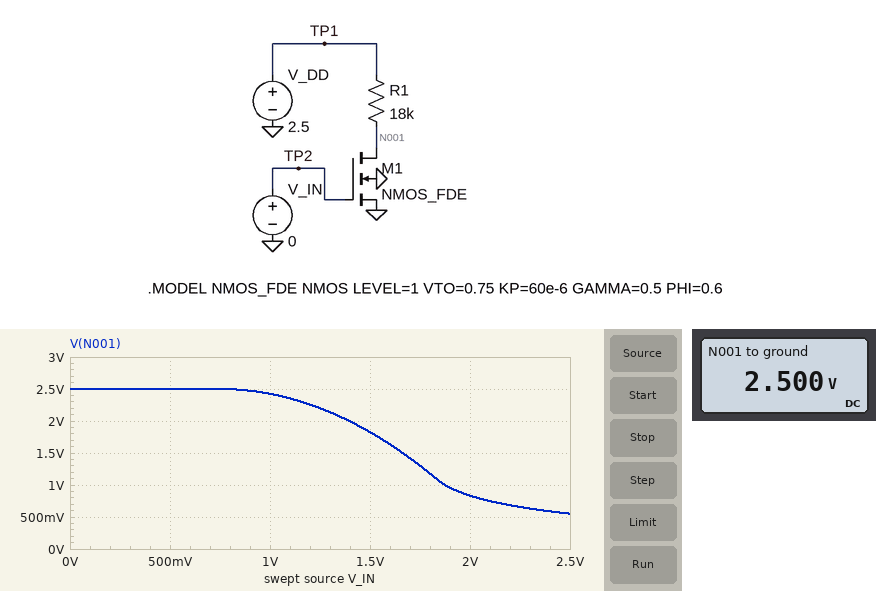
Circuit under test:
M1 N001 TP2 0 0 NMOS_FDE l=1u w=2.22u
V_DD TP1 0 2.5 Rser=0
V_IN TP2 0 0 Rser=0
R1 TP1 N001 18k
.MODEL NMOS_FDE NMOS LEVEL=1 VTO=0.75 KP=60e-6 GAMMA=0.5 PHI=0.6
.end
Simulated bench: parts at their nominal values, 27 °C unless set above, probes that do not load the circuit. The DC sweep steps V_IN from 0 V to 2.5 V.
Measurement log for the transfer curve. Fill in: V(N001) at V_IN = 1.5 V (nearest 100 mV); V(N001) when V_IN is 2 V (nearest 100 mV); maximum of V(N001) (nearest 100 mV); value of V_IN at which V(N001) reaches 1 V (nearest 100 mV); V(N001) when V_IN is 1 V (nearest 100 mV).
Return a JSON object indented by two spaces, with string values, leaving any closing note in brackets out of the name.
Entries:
{
  "V(N001) at V_IN = 1.5 V": "1.8 V",
  "V(N001) when V_IN is 2 V": "800 mV",
  "maximum of V(N001)": "2.5 V",
  "value of V_IN at which V(N001) reaches 1 V": "1.9 V",
  "V(N001) when V_IN is 1 V": "2.4 V"
}
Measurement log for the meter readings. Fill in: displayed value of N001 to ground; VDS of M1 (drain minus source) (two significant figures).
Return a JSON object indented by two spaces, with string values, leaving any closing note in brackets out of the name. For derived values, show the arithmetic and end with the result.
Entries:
{
  "displayed value of N001 to ground": "2.500 V",
  "VDS of M1 (drain minus source)": "2.5 V = 2.5 V"
}
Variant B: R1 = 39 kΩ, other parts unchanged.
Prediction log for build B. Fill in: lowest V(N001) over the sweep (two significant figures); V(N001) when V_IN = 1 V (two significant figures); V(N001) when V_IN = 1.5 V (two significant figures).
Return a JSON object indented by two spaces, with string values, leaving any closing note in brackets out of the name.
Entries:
{
  "lowest V(N001) over the sweep": "270 mV",
  "V(N001) when V_IN = 1 V": "2.3 V",
  "V(N001) when V_IN = 1.5 V": "1.0 V"
}
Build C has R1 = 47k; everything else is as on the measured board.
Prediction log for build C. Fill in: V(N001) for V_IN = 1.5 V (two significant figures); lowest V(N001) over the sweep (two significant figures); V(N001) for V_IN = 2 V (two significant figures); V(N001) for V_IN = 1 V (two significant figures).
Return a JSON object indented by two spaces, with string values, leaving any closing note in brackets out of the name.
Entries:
{
  "V(N001) for V_IN = 1.5 V": "740 mV",
  "lowest V(N001) over the sweep": "220 mV",
  "V(N001) for V_IN = 2 V": "320 mV",
  "V(N001) for V_IN = 1 V": "2.3 V"
}
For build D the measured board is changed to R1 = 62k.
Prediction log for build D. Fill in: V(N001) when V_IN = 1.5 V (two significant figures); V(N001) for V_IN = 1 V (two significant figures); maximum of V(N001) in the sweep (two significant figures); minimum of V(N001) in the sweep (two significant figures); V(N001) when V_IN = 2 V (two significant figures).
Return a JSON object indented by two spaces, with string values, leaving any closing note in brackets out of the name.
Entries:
{
  "V(N001) when V_IN = 1.5 V": "480 mV",
  "V(N001) for V_IN = 1 V": "2.2 V",
  "maximum of V(N001) in the sweep": "2.5 V",
  "minimum of V(N001) in the sweep": "170 mV",
  "V(N001) when V_IN = 2 V": "240 mV"
}
